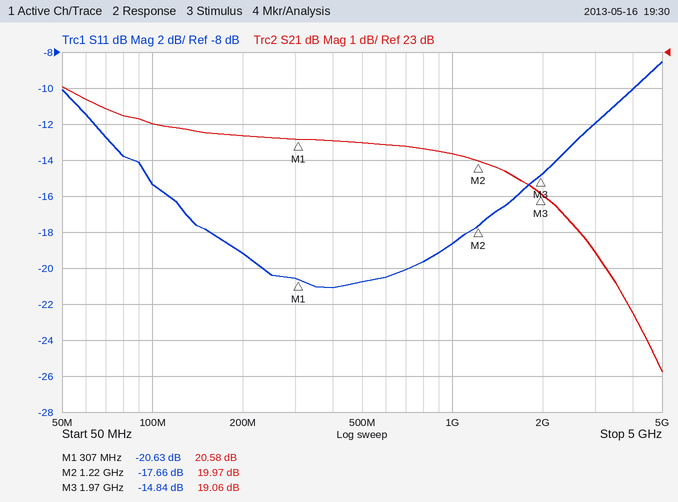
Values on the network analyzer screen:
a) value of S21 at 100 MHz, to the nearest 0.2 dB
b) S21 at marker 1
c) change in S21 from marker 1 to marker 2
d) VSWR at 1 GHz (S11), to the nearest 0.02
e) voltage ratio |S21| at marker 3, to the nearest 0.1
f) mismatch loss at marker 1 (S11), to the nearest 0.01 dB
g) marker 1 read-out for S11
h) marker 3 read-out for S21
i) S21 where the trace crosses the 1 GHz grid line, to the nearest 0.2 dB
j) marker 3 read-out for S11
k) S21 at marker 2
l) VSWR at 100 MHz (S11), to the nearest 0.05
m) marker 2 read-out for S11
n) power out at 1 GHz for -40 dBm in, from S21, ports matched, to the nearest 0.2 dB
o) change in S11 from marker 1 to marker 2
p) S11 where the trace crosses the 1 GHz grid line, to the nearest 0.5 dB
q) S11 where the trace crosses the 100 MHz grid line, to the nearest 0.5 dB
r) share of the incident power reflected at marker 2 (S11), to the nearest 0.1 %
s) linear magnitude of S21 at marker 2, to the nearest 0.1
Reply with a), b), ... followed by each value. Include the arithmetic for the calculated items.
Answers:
a) 21.0 dB
b) 20.58 dB
c) 19.97 − (20.58) = -0.61 dB
d) |Γ| = 10^(-18.5/20) = 0.1189; VSWR = (1 + 0.1189)/(1 − 0.1189) ≈ 1.27, so 1.26 to the nearest 0.02
e) 10^(19.06/20) ≈ 9.0
f) −10 log10(1 − 10^(-20.63/10)) ≈ 0.04 dB
g) -20.63 dB
h) 19.06 dB
i) 20.2 dB
j) -14.84 dB
k) 19.97 dB
l) |Γ| = 10^(-15.5/20) = 0.1679; VSWR = (1 + 0.1679)/(1 − 0.1679) ≈ 1.40
m) -17.66 dB
n) -40 dBm + (20.2 dB) = -19.8 dBm
o) -17.66 − (-20.63) = 2.97 dB
p) -18.5 dB
q) -15.5 dB
r) 10^(-17.66/10) ≈ 1.7 %
s) 10^(19.97/20) ≈ 10.0
